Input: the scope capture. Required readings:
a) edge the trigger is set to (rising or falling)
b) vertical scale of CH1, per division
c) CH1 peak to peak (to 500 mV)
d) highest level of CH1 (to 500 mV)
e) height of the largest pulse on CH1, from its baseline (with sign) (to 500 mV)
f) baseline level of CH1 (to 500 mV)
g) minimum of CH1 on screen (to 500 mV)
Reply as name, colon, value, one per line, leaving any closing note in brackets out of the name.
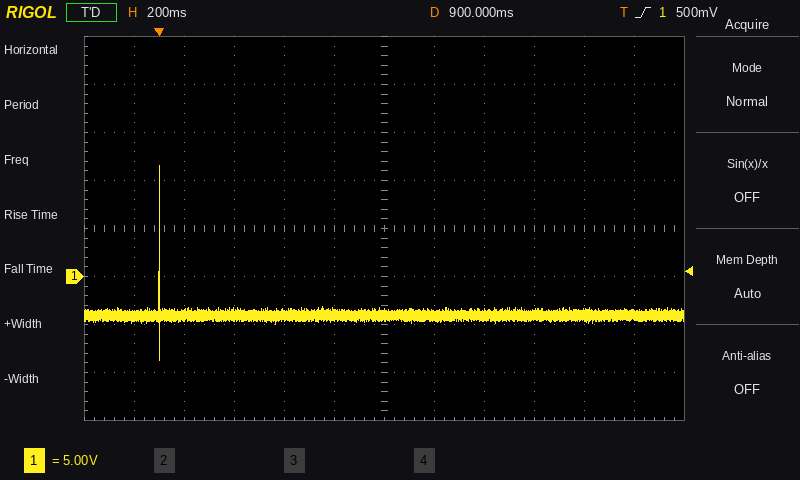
edge the trigger is set to: rising
vertical scale of CH1, per division: 5 V
CH1 peak to peak: 20.5 V
highest level of CH1: 11.5 V
height of the largest pulse on CH1, from its baseline (with sign): +15.5 V
baseline level of CH1: -4.0 V
minimum of CH1 on screen: -9.0 V
